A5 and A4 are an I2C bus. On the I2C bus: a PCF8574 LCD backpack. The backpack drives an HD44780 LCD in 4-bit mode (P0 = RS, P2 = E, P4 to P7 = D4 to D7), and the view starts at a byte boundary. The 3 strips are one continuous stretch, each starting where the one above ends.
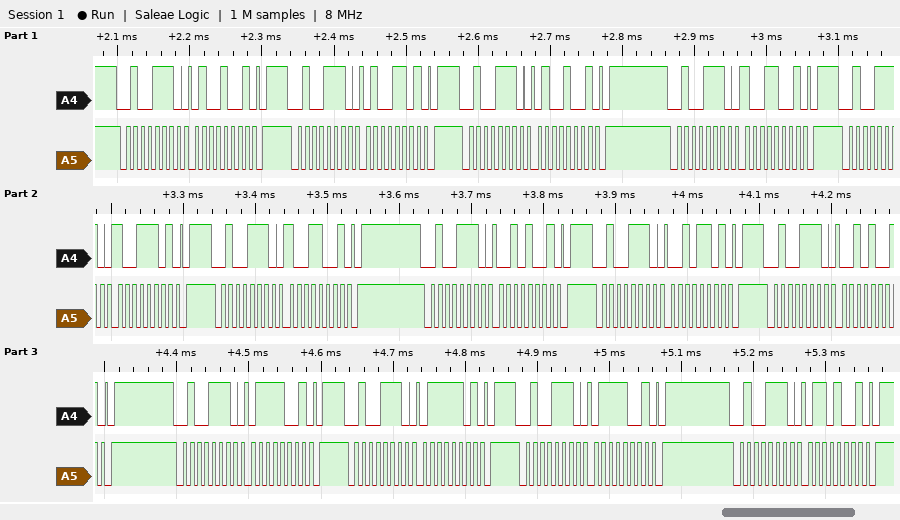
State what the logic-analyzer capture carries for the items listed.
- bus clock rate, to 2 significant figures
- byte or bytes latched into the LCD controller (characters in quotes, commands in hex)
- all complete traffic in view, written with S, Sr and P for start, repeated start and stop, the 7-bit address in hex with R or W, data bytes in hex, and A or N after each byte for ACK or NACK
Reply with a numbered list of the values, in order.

1. 100 kHz
2. 'I' '''
3. S 27W A 49 A P S 27W A 4D A P S 27W A 49 A P S 27W A 99 A P S 27W A 9D A P S 27W A 99 A P S 27W A 29 A P S 27W A 2D A P S 27W A 29 A P S 27W A 79 A P S 27W A 7D A P S 27W A 79 A P S 27W A 69 A P
